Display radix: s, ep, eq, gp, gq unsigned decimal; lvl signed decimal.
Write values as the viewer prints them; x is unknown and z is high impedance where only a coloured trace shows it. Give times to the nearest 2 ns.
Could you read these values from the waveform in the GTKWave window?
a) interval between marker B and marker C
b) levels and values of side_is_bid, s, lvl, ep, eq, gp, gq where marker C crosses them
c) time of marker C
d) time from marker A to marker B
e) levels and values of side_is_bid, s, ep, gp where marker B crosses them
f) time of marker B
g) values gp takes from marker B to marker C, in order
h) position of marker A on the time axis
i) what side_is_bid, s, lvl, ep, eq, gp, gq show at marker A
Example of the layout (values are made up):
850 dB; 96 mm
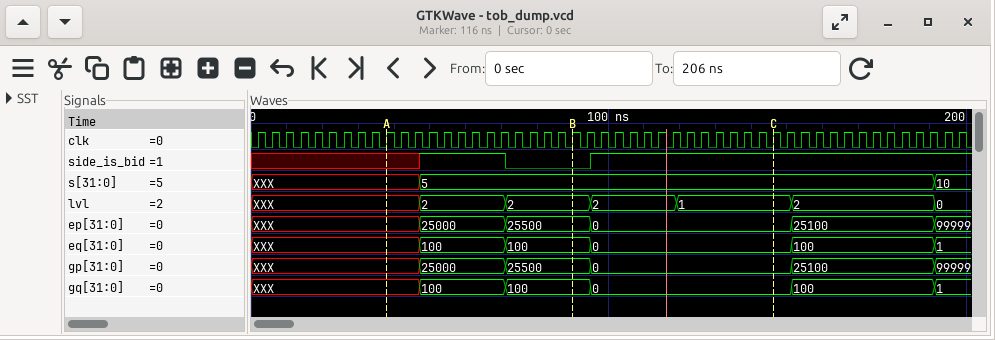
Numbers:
56 ns; side_is_bid=1, s=5, lvl=1, ep=0, eq=0, gp=0, gq=0; 146 ns; 52 ns; side_is_bid=0, s=5, ep=25500, gp=25500; 90 ns; 25500, 0; 38 ns; side_is_bid=x, s=XXX, lvl=XXX, ep=XXX, eq=XXX, gp=XXX, gq=XXX
